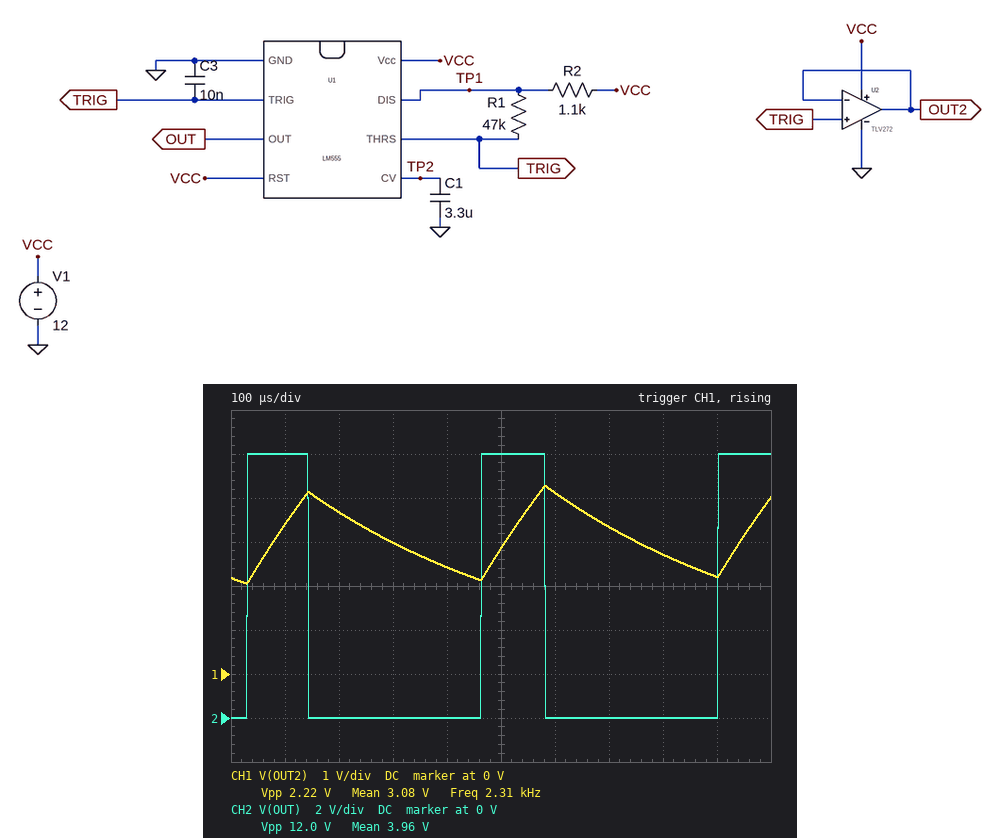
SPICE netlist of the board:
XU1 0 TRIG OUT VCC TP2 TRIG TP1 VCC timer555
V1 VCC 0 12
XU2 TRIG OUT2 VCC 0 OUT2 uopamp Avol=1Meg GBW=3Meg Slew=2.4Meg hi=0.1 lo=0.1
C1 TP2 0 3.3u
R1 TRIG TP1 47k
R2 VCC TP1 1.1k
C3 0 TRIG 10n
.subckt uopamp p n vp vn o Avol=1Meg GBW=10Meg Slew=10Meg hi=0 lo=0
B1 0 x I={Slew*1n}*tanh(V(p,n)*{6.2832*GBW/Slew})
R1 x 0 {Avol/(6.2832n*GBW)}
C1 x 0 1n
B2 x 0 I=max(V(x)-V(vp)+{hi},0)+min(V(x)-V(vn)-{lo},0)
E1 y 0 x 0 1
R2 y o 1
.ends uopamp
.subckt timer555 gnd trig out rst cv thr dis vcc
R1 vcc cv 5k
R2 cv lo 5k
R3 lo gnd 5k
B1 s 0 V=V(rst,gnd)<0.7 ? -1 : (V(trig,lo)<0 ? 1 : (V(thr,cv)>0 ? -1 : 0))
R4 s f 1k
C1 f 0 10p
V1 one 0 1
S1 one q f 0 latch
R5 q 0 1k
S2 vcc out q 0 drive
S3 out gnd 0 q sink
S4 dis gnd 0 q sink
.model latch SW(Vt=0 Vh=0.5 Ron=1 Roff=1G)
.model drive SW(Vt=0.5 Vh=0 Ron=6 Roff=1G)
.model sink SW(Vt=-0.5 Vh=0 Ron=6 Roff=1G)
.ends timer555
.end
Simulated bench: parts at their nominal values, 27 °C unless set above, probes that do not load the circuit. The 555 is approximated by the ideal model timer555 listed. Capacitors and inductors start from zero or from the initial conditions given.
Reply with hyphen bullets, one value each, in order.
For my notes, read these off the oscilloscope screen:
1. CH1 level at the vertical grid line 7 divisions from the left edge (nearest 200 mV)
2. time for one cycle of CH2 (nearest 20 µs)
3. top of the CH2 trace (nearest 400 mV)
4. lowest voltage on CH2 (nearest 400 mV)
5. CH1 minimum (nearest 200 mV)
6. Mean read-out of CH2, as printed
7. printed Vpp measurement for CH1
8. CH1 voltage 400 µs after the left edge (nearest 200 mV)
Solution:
- 3.4 V
- 440 µs
- 12.0 V
- 0 V
- 2.0 V
- 3.96 V
- 2.22 V
- 2.4 V
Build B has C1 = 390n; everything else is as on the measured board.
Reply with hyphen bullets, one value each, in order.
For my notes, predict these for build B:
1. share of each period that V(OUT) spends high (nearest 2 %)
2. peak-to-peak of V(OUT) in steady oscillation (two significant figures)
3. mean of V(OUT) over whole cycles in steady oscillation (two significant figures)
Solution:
- 50 %
- 12 V
- 6.0 V
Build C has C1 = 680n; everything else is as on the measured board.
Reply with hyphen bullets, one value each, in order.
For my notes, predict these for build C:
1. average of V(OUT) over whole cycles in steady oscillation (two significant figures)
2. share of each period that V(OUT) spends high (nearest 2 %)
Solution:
- 5.9 V
- 50 %
